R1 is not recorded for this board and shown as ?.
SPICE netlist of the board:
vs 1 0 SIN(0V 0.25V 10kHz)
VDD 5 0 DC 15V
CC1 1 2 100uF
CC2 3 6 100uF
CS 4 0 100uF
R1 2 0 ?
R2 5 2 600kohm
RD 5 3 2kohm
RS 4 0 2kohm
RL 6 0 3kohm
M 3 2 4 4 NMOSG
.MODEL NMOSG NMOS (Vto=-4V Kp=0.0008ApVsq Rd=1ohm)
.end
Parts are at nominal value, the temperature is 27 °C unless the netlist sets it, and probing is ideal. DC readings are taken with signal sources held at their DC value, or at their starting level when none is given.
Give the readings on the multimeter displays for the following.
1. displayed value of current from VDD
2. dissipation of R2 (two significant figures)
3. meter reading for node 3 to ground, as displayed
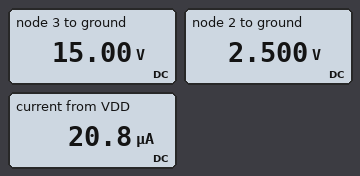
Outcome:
20.8 µA
260 µW
15.00 V
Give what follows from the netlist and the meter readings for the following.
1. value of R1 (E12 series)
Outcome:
120 kΩ
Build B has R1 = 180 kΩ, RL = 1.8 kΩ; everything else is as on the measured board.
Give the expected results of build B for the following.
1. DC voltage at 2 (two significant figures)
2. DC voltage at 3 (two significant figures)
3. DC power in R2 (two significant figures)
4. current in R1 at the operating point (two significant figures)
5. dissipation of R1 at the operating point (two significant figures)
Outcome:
3.5 V
15 V
220 µW
19 µA
67 µW
